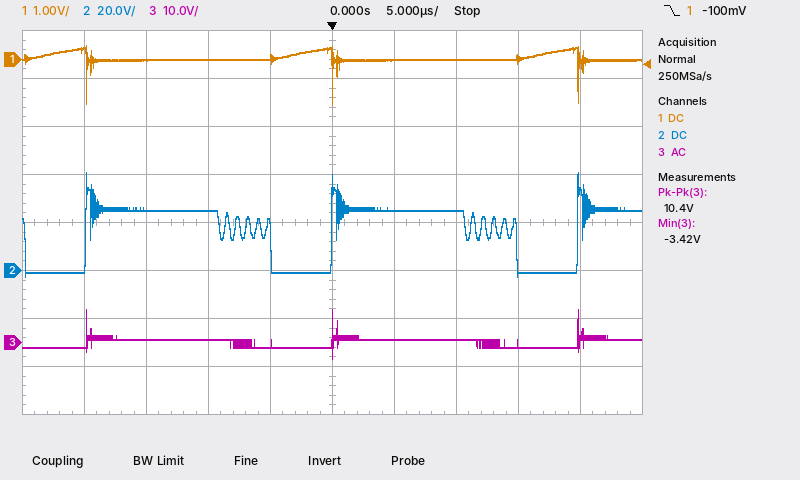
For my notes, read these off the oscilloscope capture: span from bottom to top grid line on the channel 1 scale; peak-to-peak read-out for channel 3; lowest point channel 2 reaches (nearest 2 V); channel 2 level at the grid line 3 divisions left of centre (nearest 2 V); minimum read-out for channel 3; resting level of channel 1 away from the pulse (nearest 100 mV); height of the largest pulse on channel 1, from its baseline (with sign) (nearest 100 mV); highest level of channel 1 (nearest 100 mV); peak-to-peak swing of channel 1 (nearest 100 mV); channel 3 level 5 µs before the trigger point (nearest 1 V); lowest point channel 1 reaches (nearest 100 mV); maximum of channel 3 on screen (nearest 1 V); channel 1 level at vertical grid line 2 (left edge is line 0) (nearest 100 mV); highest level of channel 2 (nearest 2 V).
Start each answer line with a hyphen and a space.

- 8 V
- 10.4 V
- -2 V
- 26 V
- -3.42 V
- 0.0 V
- -900 mV
- 300 mV
- 1.2 V
- 0 V
- -900 mV
- 7 V
- 0.0 V
- 40 V
